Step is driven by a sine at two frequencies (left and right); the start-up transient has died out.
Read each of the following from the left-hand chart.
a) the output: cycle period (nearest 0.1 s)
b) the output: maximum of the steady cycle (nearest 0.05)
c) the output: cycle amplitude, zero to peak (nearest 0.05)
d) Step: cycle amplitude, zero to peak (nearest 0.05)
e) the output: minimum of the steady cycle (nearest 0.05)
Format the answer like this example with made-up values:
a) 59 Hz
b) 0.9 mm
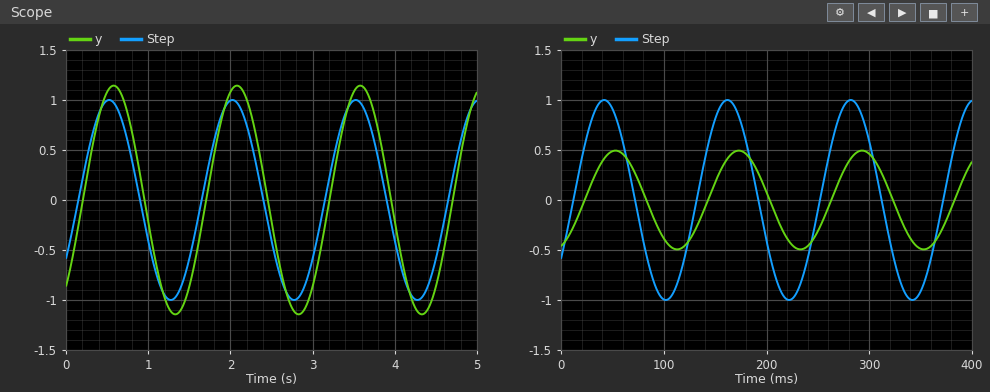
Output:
a) 1.5 s
b) 1.15
c) 1.15
d) 1.00
e) -1.15
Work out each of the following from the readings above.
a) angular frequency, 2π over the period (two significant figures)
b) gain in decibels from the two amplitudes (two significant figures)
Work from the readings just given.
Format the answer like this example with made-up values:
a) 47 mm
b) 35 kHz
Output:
a) 4.2 rad/s
b) 1.2 dB
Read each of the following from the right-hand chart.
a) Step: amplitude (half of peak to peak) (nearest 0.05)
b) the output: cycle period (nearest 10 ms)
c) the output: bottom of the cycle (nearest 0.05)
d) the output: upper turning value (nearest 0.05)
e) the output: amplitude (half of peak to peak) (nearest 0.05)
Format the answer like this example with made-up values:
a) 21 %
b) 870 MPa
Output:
a) 1.00
b) 120 ms
c) -0.50
d) 0.50
e) 0.50
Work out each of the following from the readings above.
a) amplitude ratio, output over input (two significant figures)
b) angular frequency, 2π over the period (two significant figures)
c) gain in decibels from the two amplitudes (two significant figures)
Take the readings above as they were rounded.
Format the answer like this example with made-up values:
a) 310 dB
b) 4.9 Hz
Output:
a) 0.50
b) 0.052 rad/ms
c) -6.0 dB
